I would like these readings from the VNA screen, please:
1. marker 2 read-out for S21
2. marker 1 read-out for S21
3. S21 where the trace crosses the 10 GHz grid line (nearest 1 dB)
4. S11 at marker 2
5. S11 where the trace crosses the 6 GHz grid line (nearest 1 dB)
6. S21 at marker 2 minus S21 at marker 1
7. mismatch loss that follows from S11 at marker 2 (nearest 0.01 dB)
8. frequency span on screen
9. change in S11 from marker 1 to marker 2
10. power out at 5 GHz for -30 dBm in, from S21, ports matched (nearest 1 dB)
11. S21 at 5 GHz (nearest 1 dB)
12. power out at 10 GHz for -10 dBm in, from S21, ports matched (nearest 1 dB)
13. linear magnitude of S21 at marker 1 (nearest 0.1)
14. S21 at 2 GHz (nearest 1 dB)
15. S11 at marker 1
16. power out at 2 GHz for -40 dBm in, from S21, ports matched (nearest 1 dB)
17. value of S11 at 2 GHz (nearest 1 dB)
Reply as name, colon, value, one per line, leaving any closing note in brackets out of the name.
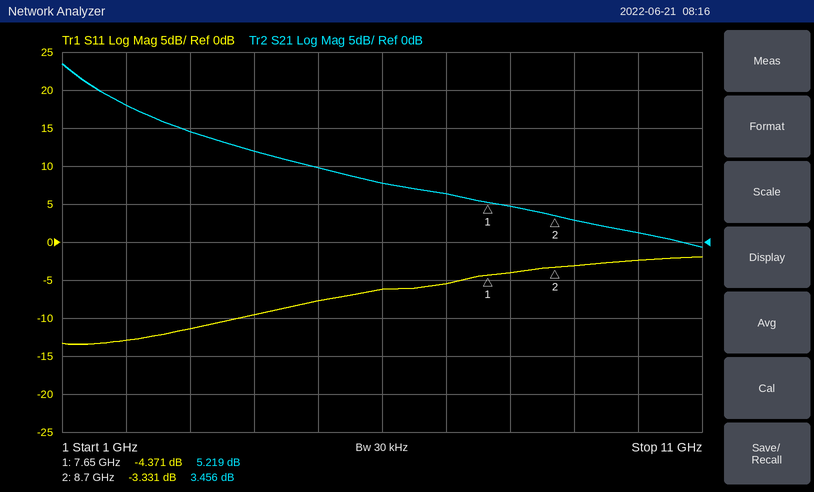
marker 2 read-out for S21: 3.456 dB
marker 1 read-out for S21: 5.219 dB
S21 where the trace crosses the 10 GHz grid line: 1 dB
S11 at marker 2: -3.331 dB
S11 where the trace crosses the 6 GHz grid line: -6 dB
S21 at marker 2 minus S21 at marker 1: -1.763 dB
mismatch loss that follows from S11 at marker 2: 2.71 dB
frequency span on screen: 10 GHz
change in S11 from marker 1 to marker 2: 1.040 dB
power out at 5 GHz for -30 dBm in, from S21, ports matched: -20 dBm
S21 at 5 GHz: 10 dB
power out at 10 GHz for -10 dBm in, from S21, ports matched: -9 dBm
linear magnitude of S21 at marker 1: 1.8
S21 at 2 GHz: 18 dB
S11 at marker 1: -4.371 dB
power out at 2 GHz for -40 dBm in, from S21, ports matched: -22 dBm
value of S11 at 2 GHz: -13 dB
